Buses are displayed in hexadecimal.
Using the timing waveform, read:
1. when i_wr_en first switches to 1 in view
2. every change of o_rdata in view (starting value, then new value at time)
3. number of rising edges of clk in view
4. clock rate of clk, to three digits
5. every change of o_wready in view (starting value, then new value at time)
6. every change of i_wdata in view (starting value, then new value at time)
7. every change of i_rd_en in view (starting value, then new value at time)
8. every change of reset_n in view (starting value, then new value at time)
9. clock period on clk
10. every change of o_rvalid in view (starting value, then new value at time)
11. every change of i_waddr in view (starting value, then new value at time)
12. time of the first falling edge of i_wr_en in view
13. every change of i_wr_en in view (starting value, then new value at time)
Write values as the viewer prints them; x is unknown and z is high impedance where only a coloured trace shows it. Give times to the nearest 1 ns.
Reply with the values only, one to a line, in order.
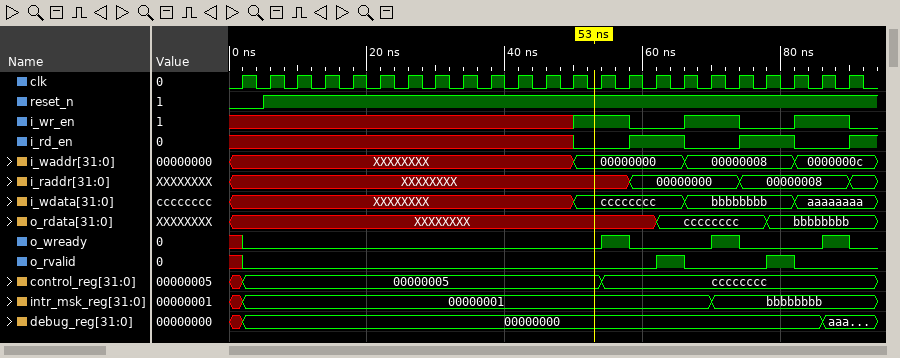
50 ns
XXXXXXXX, cccccccc at 62 ns, bbbbbbbb at 78 ns
23
250 MHz
x, 0 at 2 ns, 1 at 54 ns, 0 at 58 ns, 1 at 70 ns, 0 at 74 ns, 1 at 86 ns, 0 at 90 ns
XXXXXXXX, cccccccc at 50 ns, bbbbbbbb at 66 ns, aaaaaaaa at 82 ns
x, 0 at 50 ns, 1 at 58 ns, 0 at 66 ns, 1 at 74 ns, 0 at 82 ns, 1 at 90 ns
0, 1 at 5 ns
4 ns
x, 0 at 2 ns, 1 at 62 ns, 0 at 66 ns, 1 at 78 ns, 0 at 82 ns
XXXXXXXX, 00000000 at 50 ns, 00000008 at 66 ns, 0000000c at 82 ns
58 ns
x, 1 at 50 ns, 0 at 58 ns, 1 at 66 ns, 0 at 74 ns, 1 at 82 ns, 0 at 90 ns
